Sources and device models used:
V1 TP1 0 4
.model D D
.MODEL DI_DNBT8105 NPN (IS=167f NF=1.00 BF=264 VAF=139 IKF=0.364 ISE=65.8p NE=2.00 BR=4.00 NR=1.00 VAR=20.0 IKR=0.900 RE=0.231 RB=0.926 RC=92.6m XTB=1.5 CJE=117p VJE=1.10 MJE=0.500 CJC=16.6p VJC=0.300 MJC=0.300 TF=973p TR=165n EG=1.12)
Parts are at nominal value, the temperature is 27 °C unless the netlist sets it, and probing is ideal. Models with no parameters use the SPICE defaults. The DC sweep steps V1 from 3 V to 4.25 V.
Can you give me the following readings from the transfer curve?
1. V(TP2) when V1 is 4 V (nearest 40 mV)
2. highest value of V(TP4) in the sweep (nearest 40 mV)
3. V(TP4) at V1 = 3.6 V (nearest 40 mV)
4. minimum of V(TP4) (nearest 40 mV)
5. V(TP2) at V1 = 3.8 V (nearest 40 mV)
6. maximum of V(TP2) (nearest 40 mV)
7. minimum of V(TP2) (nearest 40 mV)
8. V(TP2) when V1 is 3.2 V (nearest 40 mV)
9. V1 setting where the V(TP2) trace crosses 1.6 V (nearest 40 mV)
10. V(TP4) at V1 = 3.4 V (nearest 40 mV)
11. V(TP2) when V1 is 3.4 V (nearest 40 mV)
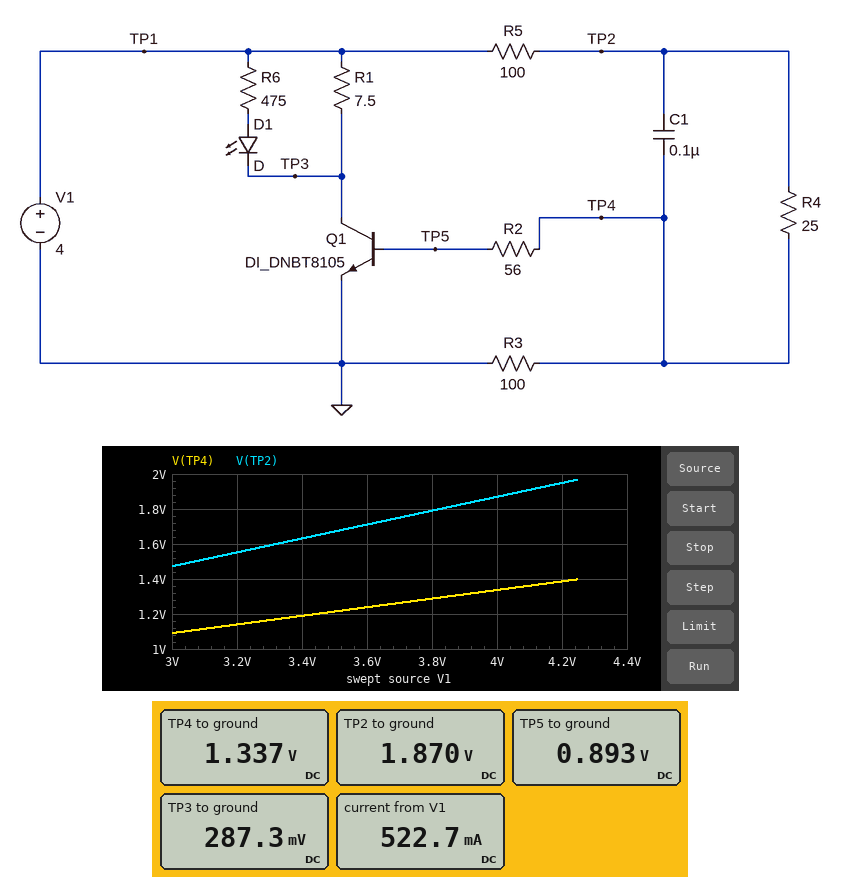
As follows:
1.88 V
1.40 V
1.24 V
1.08 V
1.80 V
1.96 V
1.48 V
1.56 V
3.32 V
1.20 V
1.64 V
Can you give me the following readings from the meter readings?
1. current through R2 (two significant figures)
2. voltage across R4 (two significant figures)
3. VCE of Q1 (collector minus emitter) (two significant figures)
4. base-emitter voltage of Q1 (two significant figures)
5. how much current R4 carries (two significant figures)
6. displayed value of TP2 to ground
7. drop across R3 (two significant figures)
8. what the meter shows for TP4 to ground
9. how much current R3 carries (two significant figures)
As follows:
7.9 mA
530 mV
290 mV
890 mV
21 mA
1.870 V
1.3 V
1.337 V
13 mA
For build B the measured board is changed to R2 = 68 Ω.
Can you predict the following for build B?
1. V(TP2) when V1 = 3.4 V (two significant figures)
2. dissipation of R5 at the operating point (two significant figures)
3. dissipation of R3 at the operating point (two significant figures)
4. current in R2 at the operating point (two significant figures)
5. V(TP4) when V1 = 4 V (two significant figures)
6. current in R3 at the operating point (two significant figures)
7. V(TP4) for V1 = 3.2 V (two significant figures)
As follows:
1.7 V
44 mW
19 mW
7.2 mA
1.4 V
14 mA
1.2 V
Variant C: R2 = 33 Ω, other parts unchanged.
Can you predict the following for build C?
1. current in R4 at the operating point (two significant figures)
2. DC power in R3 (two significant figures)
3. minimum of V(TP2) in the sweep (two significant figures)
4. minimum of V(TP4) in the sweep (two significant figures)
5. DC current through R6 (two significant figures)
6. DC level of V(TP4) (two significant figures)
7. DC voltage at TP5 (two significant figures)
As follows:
22 mA
15 mW
1.4 V
1.0 V
6.4 mA
1.2 V
900 mV
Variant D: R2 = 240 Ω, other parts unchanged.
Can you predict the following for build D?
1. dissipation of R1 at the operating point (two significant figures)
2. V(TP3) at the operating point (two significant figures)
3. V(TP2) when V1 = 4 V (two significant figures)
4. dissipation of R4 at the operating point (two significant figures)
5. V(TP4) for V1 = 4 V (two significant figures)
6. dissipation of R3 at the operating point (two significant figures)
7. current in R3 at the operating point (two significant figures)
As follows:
1.0 W
1.2 V
2.1 V
9.2 mW
1.6 V
26 mW
16 mA
